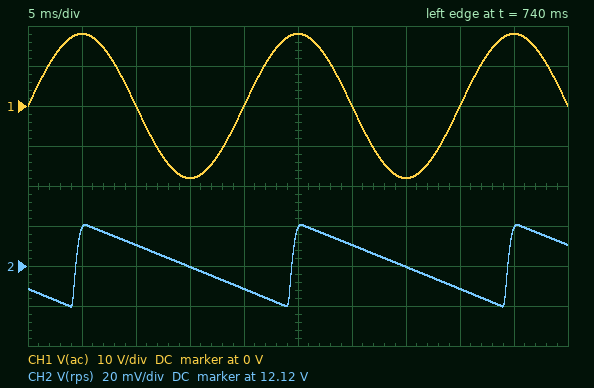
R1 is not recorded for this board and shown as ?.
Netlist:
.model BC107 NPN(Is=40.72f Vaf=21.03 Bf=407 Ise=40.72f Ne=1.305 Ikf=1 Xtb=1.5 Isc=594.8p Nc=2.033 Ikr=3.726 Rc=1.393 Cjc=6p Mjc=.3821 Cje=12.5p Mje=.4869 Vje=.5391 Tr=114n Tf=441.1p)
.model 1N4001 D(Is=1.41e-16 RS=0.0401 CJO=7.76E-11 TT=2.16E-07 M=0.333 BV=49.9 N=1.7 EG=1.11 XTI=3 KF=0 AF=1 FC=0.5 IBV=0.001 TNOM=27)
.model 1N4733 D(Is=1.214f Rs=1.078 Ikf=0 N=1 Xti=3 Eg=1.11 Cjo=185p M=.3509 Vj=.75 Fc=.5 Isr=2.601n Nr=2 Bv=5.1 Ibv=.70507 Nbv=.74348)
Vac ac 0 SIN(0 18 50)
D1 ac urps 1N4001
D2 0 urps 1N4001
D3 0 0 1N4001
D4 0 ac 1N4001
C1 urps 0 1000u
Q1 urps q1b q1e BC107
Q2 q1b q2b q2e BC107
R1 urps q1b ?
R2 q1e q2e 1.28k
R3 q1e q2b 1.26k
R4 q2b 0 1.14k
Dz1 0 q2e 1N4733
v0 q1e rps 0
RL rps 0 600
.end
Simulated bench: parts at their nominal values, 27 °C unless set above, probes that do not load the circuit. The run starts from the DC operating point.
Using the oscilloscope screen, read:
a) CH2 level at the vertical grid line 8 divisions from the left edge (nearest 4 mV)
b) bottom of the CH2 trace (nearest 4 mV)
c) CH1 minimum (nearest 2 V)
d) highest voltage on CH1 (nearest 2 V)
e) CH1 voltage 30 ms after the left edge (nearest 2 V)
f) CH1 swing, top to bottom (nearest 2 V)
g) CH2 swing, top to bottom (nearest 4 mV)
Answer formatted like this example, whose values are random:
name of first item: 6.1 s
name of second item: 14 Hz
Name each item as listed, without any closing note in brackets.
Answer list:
CH2 level at the vertical grid line 8 divisions from the left edge: 12.108 V
bottom of the CH2 trace: 12.100 V
CH1 minimum: -18 V
highest voltage on CH1: 18 V
CH1 voltage 30 ms after the left edge: 0 V
CH1 swing, top to bottom: 36 V
CH2 swing, top to bottom: 40 mV
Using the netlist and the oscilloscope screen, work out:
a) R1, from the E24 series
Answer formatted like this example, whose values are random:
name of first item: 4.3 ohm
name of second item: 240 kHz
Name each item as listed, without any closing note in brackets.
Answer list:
R1, from the E24 series: 240 Ω
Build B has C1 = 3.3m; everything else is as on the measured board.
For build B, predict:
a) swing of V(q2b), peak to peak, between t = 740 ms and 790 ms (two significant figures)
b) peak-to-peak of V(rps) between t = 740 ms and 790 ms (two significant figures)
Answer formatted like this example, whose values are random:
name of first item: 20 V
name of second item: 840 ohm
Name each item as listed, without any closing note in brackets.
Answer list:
swing of V(q2b), peak to peak, between t = 740 ms and 790 ms: 4.0 mV
peak-to-peak of V(rps) between t = 740 ms and 790 ms: 12 mV
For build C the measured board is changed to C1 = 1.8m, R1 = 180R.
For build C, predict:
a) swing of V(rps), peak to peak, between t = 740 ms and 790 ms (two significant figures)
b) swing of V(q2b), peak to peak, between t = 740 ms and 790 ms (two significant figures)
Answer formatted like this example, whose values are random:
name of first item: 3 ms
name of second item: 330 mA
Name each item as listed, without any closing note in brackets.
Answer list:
swing of V(rps), peak to peak, between t = 740 ms and 790 ms: 29 mV
swing of V(q2b), peak to peak, between t = 740 ms and 790 ms: 9.0 mV
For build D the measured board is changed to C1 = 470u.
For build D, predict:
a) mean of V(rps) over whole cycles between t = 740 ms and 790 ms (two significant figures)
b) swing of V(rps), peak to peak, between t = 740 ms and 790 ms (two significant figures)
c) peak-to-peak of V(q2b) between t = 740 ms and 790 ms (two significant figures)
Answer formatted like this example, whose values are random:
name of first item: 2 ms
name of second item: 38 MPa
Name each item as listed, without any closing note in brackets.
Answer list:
mean of V(rps) over whole cycles between t = 740 ms and 790 ms: 12 V
swing of V(rps), peak to peak, between t = 740 ms and 790 ms: 88 mV
peak-to-peak of V(q2b) between t = 740 ms and 790 ms: 29 mV
